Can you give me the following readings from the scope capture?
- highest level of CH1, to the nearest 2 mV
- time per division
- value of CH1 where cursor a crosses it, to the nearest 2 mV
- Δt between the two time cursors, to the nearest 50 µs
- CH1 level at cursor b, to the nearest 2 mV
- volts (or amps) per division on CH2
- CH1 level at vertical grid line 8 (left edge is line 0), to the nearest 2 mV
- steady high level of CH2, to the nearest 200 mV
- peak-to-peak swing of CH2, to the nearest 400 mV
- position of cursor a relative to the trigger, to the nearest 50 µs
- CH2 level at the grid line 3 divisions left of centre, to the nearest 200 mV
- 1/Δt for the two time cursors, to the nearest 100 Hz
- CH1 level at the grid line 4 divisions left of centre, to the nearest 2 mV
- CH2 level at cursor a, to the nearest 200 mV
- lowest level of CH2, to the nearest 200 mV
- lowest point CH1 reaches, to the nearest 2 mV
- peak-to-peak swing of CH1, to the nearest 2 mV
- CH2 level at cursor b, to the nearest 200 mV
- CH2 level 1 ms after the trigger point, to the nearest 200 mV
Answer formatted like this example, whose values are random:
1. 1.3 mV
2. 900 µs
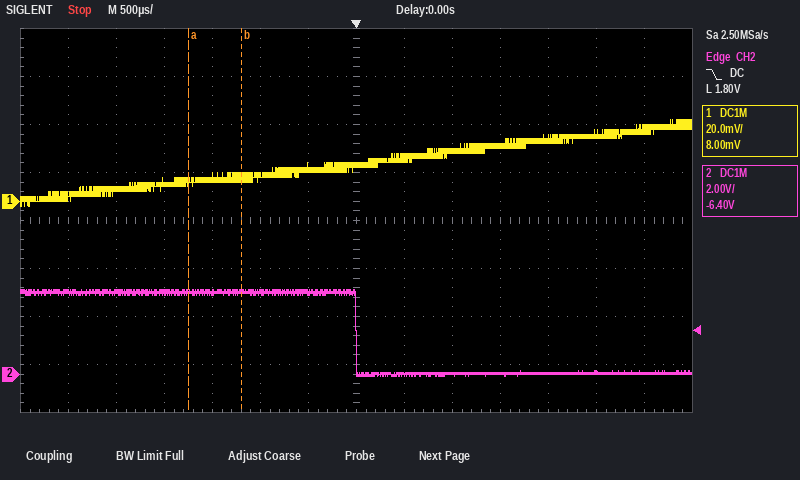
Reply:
1. 34 mV
2. 500 µs
3. 8 mV
4. 550 µs
5. 10 mV
6. 2 V
7. 18 mV
8. 3.4 V
9. 3.6 V
10. -1.75 ms
11. 3.4 V
12. 1.8 kHz
13. 8 mV
14. 3.4 V
15. 0.0 V
16. -2 mV
17. 36 mV
18. 3.4 V
19. 0.0 V
